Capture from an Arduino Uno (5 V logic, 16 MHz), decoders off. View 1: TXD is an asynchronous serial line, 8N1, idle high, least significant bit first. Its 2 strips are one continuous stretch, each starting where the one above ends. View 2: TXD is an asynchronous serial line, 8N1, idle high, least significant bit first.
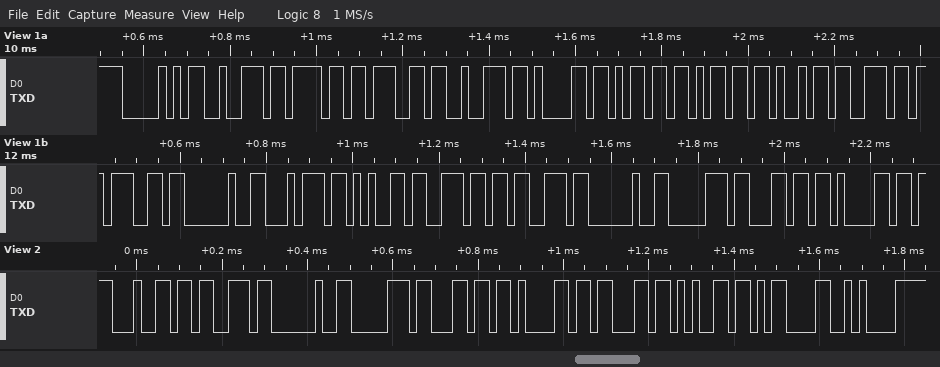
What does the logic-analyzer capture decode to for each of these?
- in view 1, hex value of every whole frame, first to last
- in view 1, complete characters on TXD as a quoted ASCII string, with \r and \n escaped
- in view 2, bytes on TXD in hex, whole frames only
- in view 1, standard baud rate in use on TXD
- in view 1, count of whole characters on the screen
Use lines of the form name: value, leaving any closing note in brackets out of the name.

in view 1, hex value of every whole frame, first to last: 50 72 6F 67 72 61 6D 6D 69 6E 67 20 74 65 6E 73 20 70 6C 61
in view 1, complete characters on TXD as a quoted ASCII string, with \r and \n escaped: "Programming tens pla"
in view 2, bytes on TXD in hex, whole frames only: 64 73 20 70 6C 61 63 65 0D 0A
in view 1, standard baud rate in use on TXD: 57600 baud
in view 1, count of whole characters on the screen: 20
